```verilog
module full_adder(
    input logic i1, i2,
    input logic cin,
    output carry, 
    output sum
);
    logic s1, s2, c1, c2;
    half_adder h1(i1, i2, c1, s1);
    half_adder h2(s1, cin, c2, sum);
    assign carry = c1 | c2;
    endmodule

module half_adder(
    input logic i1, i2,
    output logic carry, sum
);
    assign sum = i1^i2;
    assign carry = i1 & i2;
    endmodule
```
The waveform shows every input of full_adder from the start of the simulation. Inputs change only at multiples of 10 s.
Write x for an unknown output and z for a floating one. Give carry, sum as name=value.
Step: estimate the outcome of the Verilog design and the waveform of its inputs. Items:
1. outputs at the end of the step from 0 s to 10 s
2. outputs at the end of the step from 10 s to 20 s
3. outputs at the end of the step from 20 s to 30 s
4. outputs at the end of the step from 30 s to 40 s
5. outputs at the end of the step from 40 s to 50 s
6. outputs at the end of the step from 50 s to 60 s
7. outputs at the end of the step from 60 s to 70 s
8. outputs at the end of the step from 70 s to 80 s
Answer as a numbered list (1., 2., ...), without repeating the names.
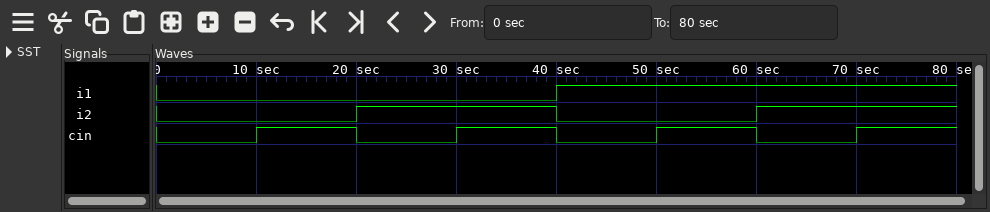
1. carry=0, sum=0
2. carry=0, sum=1
3. carry=0, sum=1
4. carry=1, sum=0
5. carry=0, sum=1
6. carry=1, sum=0
7. carry=1, sum=0
8. carry=1, sum=1
